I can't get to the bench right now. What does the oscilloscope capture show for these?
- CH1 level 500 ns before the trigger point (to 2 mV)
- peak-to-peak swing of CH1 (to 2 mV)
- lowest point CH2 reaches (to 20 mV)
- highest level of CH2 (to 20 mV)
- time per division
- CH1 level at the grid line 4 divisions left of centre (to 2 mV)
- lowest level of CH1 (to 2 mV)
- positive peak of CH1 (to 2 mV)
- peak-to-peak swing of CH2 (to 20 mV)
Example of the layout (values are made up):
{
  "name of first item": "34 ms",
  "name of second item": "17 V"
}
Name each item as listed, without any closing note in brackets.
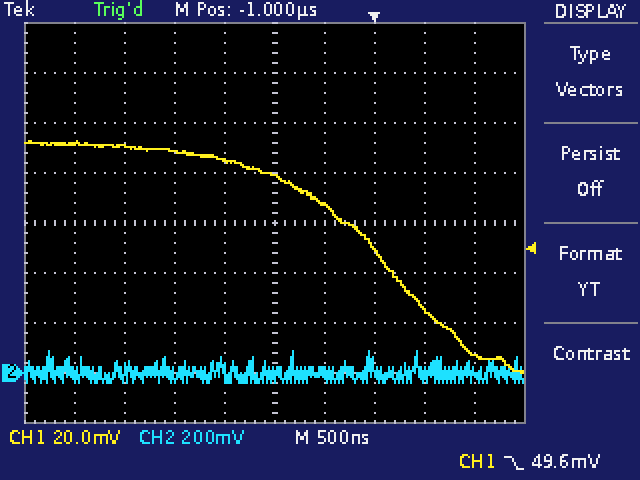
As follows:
{
  "CH1 level 500 ns before the trigger point": "68 mV",
  "peak-to-peak swing of CH1": "92 mV",
  "lowest point CH2 reaches": "-40 mV",
  "highest level of CH2": "80 mV",
  "time per division": "500 ns",
  "CH1 level at the grid line 4 divisions left of centre": "92 mV",
  "lowest level of CH1": "0 mV",
  "positive peak of CH1": "92 mV",
  "peak-to-peak swing of CH2": "120 mV"
}
